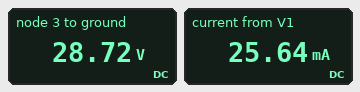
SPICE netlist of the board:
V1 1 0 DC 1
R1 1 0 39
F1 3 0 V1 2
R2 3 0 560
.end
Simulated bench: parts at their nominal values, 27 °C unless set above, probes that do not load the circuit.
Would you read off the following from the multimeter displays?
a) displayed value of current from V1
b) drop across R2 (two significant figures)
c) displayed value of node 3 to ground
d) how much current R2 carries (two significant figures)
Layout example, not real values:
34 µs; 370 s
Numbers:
25.64 mA; 29 V; 28.72 V; 51 mA
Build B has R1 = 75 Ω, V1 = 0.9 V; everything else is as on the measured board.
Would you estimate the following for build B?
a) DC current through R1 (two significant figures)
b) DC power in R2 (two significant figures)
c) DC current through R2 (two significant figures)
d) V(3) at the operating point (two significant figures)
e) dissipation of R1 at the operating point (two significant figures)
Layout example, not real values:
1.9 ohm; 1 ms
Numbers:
12 mA; 320 mW; 24 mA; 13 V; 11 mW
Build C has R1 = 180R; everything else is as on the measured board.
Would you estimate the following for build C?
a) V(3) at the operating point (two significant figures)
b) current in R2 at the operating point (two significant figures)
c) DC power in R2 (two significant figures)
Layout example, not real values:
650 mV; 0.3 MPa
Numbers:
6.2 V; 11 mA; 69 mW
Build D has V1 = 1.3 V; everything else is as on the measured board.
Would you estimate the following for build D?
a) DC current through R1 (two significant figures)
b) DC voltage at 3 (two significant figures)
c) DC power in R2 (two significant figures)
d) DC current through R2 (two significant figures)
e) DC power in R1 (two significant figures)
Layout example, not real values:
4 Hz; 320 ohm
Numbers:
33 mA; 37 V; 2.5 W; 67 mA; 43 mW
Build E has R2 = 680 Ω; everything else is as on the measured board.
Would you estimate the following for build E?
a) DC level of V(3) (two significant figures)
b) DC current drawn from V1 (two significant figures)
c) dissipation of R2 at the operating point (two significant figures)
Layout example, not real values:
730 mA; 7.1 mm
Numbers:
35 V; 26 mA; 1.8 W
